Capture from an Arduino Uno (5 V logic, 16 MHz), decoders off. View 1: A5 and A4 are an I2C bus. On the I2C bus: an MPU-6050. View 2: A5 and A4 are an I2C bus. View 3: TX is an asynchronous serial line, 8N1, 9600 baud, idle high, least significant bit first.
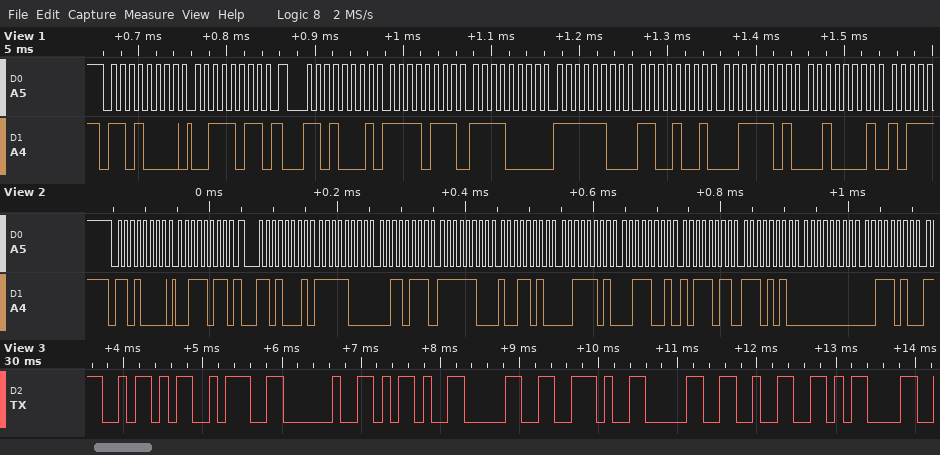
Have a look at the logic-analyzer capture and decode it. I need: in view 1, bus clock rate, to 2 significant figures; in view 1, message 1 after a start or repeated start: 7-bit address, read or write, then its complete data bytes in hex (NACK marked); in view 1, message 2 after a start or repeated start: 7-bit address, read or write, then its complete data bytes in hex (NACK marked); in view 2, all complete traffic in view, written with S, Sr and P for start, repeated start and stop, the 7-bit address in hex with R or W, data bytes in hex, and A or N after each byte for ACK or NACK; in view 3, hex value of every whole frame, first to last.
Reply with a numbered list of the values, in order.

1. 100 kHz
2. 0x68 write: 3B
3. 0x68 read: F7 F0 FC C9 3D 21
4. S 68W A 3B A Sr 68R A F8 A 37 A FC A 9A A 3D A 39 A BB A EA A 00 A 3A A
5. 5A 3A 20 2D 30 2E 30 32 0D
